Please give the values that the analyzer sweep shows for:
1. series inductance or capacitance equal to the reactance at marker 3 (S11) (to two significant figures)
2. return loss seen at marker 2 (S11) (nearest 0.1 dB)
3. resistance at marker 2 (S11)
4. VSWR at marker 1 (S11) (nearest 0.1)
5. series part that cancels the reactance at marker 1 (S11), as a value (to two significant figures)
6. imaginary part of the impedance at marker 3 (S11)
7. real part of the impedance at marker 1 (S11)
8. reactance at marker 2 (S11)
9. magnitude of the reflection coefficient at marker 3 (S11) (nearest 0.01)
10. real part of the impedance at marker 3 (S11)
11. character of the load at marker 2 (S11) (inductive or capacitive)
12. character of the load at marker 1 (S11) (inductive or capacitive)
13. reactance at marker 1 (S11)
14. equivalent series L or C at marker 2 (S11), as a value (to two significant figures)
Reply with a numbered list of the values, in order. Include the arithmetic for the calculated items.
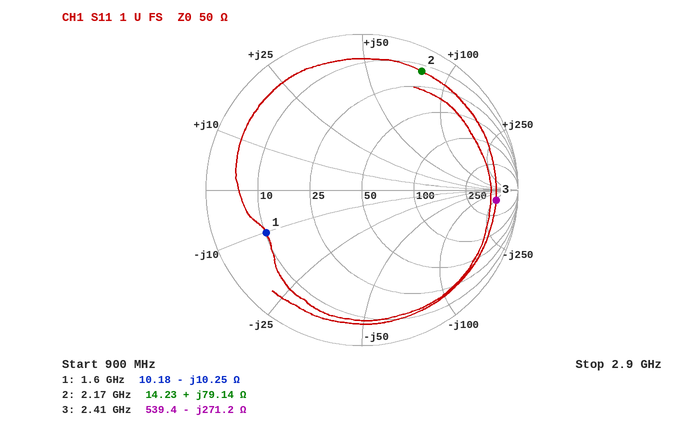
1. C = 1/(2π × 2.41 GHz × 271.2 Ω) ≈ 244 fF, so 240 fF to two significant figures
2. 1.4 dB
3. 14.23 Ω
4. 5.1
5. L = 10.25 Ω/(2π × 1.6 GHz) ≈ 1.0 nH
6. -271.2 Ω
7. 10.18 Ω
8. +79.14 Ω
9. 0.86
10. 539.4 Ω
11. inductive
12. capacitive
13. -10.25 Ω
14. L = 79.14 Ω/(2π × 2.17 GHz) ≈ 5.8 nH
